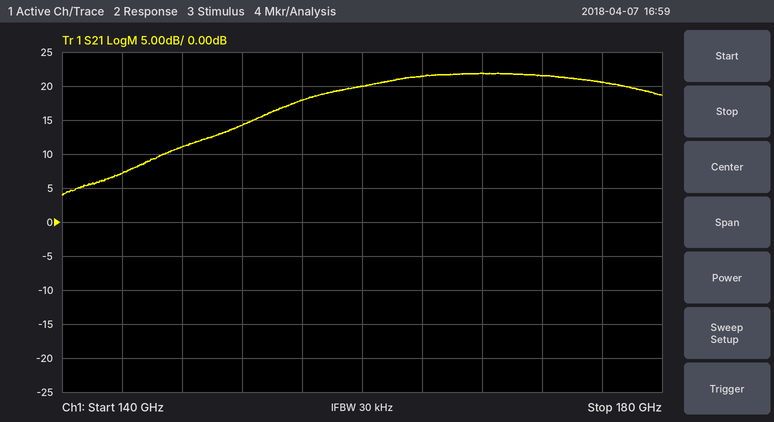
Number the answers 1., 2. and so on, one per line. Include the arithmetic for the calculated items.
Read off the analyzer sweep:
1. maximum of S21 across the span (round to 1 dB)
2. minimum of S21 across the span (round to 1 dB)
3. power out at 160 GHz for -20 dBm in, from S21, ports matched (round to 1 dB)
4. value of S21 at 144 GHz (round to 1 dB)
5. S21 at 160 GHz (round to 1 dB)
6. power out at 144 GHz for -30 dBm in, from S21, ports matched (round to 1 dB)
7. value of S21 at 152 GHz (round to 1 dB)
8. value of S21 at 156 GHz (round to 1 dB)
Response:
1. 22 dB
2. 4 dB
3. -20 dBm + (20 dB) = 0 dBm
4. 7 dB
5. 20 dB
6. -30 dBm + (7 dB) = -23 dBm
7. 14 dB
8. 18 dB
